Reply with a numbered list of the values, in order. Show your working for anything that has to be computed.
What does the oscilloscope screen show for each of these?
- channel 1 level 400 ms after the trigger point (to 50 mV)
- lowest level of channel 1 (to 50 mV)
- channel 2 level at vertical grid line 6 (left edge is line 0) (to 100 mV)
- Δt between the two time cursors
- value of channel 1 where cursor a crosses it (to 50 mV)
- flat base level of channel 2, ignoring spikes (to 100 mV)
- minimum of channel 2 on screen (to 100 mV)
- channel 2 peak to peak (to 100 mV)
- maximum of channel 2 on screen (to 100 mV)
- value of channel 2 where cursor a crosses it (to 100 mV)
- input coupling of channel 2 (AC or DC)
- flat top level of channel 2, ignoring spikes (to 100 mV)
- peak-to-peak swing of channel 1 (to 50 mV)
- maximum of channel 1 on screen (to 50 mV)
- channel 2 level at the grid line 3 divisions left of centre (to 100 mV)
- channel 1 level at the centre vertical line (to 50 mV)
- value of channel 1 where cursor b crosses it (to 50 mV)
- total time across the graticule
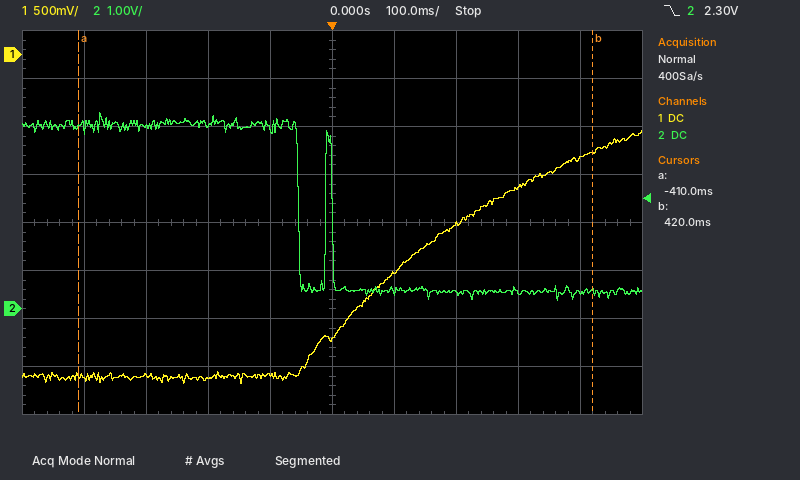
1. -1.10 V
2. -3.45 V
3. 400 mV
4. 420 ms − (-410 ms) = 830 ms
5. -3.35 V
6. 400 mV
7. 200 mV
8. 4.1 V − (200 mV) = 3.9 V
9. 4.1 V
10. 3.8 V
11. DC
12. 3.8 V
13. -800 mV − (-3.45 V) = 2.65 V
14. -800 mV
15. 3.8 V
16. -2.95 V
17. -1.00 V
18. 1 s
